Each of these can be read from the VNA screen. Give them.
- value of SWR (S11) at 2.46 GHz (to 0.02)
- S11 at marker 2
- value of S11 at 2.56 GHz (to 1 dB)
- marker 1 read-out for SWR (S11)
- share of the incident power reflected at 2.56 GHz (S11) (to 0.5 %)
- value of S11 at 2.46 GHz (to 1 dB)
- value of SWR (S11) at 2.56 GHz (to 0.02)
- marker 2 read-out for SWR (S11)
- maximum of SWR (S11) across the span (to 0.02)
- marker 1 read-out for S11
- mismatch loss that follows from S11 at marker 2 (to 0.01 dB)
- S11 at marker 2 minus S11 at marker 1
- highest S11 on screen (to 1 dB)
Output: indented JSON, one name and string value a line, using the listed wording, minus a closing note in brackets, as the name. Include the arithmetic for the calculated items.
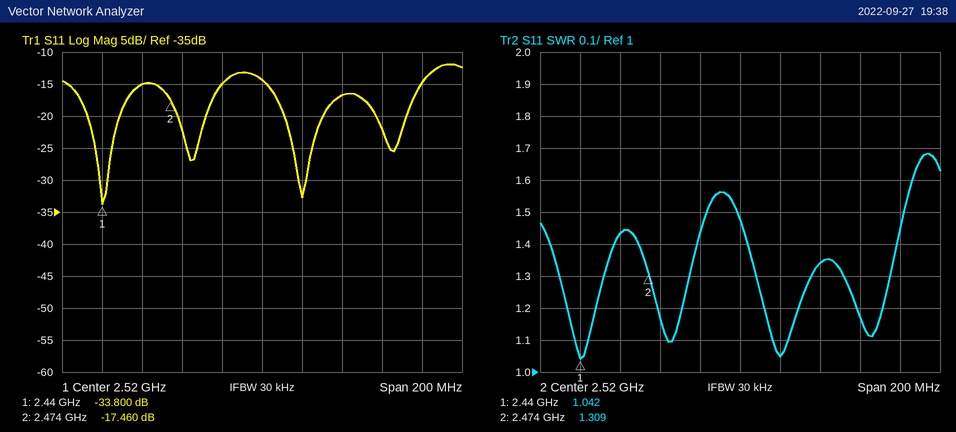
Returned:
{
  "value of SWR (S11) at 2.46 GHz": "1.44",
  "S11 at marker 2": "-17.460 dB",
  "value of S11 at 2.56 GHz": "-17 dB",
  "marker 1 read-out for SWR": "1.042",
  "share of the incident power reflected at 2.56 GHz (S11)": "10^(-17/10) ≈ 2.0 %",
  "value of S11 at 2.46 GHz": "-15 dB",
  "value of SWR (S11) at 2.56 GHz": "1.34",
  "marker 2 read-out for SWR": "1.309",
  "maximum of SWR (S11) across the span": "1.68",
  "marker 1 read-out for S11": "-33.800 dB",
  "mismatch loss that follows from S11 at marker 2": "−10 log10(1 − 10^(-17.46/10)) ≈ 0.08 dB",
  "S11 at marker 2 minus S11 at marker 1": "-17.46 − (-33.8) = 16.340 dB",
  "highest S11 on screen": "-12 dB"
}
